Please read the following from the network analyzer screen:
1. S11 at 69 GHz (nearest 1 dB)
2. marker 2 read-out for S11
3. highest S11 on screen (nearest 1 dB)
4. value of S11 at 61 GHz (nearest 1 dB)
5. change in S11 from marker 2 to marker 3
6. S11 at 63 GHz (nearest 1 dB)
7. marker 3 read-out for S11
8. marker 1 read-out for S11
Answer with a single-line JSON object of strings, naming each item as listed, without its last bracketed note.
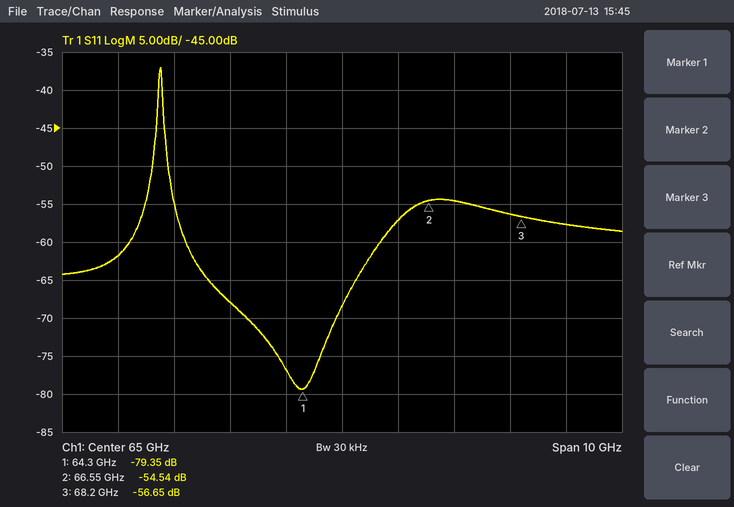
{"S11 at 69 GHz": "-58 dB", "marker 2 read-out for S11": "-54.54 dB", "highest S11 on screen": "-37 dB", "value of S11 at 61 GHz": "-62 dB", "change in S11 from marker 2 to marker 3": "-2.11 dB", "S11 at 63 GHz": "-68 dB", "marker 3 read-out for S11": "-56.65 dB", "marker 1 read-out for S11": "-79.35 dB"}
